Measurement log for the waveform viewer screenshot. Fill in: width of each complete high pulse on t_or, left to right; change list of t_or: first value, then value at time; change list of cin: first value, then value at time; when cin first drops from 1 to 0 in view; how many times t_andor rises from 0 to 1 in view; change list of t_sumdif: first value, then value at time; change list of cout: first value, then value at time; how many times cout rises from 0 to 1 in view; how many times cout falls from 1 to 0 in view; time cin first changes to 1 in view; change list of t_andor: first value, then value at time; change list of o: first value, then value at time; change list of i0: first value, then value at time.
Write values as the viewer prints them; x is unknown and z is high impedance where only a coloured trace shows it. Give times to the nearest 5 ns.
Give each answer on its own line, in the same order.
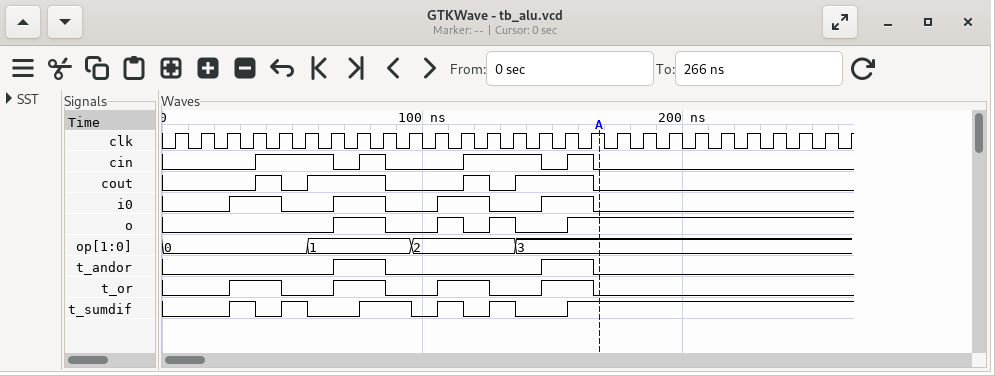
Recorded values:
20 ns, 20 ns, 20 ns, 20 ns
0, 1 at 25 ns, 0 at 45 ns, 1 at 65 ns, 0 at 85 ns, 1 at 105 ns, 0 at 125 ns, 1 at 145 ns, 0 at 165 ns
0, 1 at 35 ns, 0 at 65 ns, 1 at 75 ns, 0 at 85 ns, 1 at 115 ns, 0 at 145 ns, 1 at 155 ns, 0 at 165 ns
65 ns
2
0, 1 at 25 ns, 0 at 35 ns, 1 at 45 ns, 0 at 55 ns, 1 at 75 ns, 0 at 95 ns, 1 at 105 ns, 0 at 115 ns, 1 at 125 ns, 0 at 135 ns, 1 at 155 ns
0, 1 at 35 ns, 0 at 45 ns, 1 at 55 ns, 0 at 85 ns, 1 at 115 ns, 0 at 125 ns, 1 at 135 ns, 0 at 165 ns
4
4
35 ns
0, 1 at 65 ns, 0 at 85 ns, 1 at 145 ns, 0 at 165 ns
0, 1 at 65 ns, 0 at 85 ns, 1 at 105 ns, 0 at 115 ns, 1 at 125 ns, 0 at 135 ns, 1 at 155 ns
0, 1 at 25 ns, 0 at 45 ns, 1 at 65 ns, 0 at 85 ns, 1 at 105 ns, 0 at 125 ns, 1 at 145 ns, 0 at 165 ns
